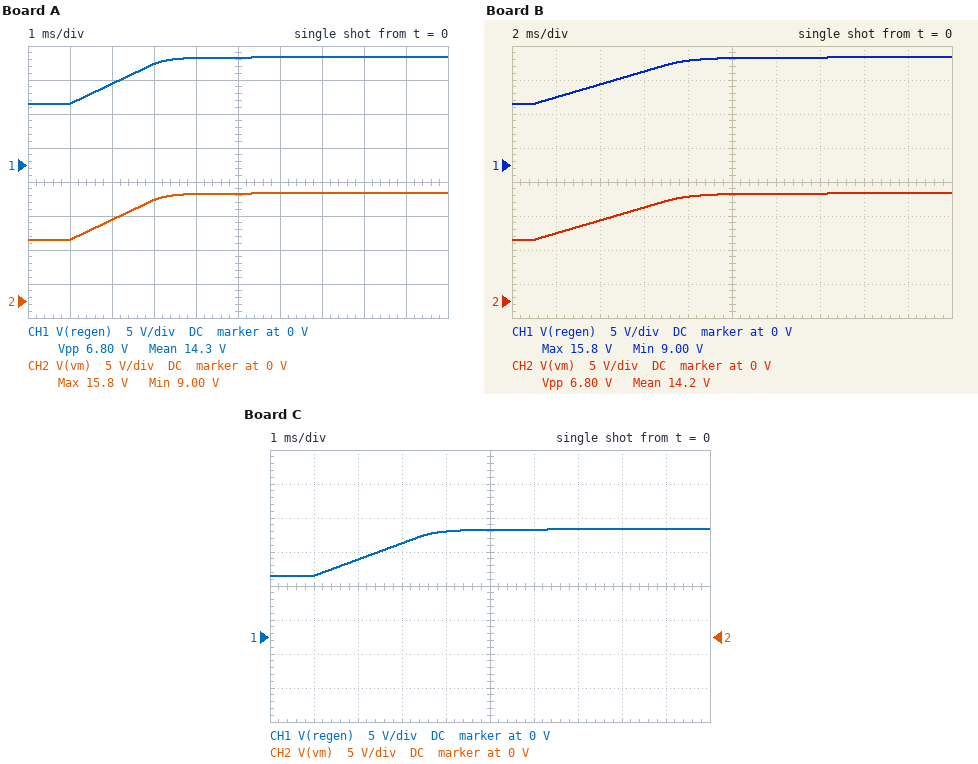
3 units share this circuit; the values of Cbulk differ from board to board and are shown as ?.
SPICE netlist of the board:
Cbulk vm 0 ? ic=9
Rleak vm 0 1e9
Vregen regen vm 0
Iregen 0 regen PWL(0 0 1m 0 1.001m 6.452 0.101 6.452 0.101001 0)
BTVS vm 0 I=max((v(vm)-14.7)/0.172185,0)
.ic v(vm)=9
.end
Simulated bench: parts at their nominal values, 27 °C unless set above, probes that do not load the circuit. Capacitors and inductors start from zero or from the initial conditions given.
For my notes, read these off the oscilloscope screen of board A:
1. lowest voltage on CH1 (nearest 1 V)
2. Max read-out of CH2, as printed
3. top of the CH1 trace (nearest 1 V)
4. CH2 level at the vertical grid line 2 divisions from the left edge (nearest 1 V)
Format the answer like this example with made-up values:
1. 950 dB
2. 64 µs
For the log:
1. 9 V
2. 15.8 V
3. 16 V
4. 12 V
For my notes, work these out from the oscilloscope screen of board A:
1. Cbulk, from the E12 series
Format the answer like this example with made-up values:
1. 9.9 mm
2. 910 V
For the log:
1. 2.2 mF
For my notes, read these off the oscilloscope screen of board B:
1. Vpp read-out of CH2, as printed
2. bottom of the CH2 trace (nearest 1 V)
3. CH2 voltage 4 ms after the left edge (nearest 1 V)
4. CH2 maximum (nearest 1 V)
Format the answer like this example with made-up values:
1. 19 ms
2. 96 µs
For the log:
1. 6.80 V
2. 9 V
3. 12 V
4. 16 V
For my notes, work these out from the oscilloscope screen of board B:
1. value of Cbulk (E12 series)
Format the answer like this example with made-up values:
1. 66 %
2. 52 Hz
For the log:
1. 6.8 mF
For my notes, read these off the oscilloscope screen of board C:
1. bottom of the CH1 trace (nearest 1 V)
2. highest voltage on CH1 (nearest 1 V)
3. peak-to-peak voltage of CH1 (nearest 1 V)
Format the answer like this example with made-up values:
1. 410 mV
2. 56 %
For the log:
1. 9 V
2. 16 V
3. 7 V
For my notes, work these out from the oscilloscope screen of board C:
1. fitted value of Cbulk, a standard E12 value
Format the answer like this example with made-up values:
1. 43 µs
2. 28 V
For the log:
1. 2.7 mF
